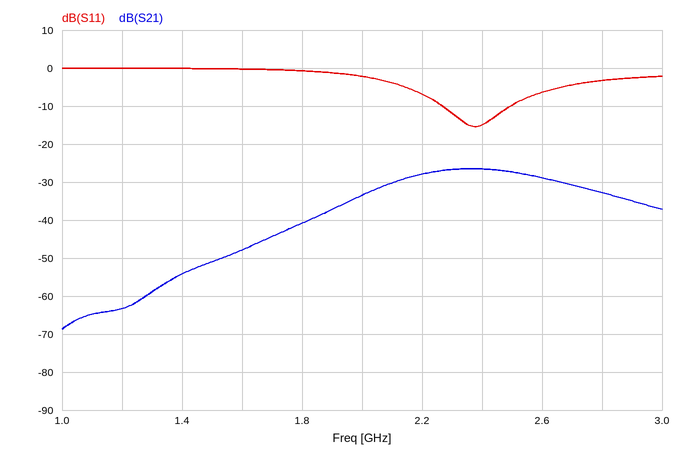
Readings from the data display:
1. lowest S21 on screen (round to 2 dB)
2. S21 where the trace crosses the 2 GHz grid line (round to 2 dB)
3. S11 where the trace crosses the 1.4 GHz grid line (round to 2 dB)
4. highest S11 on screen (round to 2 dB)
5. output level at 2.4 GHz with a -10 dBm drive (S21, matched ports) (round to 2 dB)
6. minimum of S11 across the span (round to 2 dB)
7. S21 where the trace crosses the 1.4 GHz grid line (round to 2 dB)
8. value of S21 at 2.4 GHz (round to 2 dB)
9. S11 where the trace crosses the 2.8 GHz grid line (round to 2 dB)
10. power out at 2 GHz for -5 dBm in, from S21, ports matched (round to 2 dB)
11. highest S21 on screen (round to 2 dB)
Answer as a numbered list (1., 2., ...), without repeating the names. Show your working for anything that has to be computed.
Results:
1. -68 dB
2. -34 dB
3. 0 dB
4. 0 dB
5. -10 dBm + (-26 dB) = -36 dBm
6. -16 dB
7. -54 dB
8. -26 dB
9. -4 dB
10. -5 dBm + (-34 dB) = -38 dBm
11. -26 dB
